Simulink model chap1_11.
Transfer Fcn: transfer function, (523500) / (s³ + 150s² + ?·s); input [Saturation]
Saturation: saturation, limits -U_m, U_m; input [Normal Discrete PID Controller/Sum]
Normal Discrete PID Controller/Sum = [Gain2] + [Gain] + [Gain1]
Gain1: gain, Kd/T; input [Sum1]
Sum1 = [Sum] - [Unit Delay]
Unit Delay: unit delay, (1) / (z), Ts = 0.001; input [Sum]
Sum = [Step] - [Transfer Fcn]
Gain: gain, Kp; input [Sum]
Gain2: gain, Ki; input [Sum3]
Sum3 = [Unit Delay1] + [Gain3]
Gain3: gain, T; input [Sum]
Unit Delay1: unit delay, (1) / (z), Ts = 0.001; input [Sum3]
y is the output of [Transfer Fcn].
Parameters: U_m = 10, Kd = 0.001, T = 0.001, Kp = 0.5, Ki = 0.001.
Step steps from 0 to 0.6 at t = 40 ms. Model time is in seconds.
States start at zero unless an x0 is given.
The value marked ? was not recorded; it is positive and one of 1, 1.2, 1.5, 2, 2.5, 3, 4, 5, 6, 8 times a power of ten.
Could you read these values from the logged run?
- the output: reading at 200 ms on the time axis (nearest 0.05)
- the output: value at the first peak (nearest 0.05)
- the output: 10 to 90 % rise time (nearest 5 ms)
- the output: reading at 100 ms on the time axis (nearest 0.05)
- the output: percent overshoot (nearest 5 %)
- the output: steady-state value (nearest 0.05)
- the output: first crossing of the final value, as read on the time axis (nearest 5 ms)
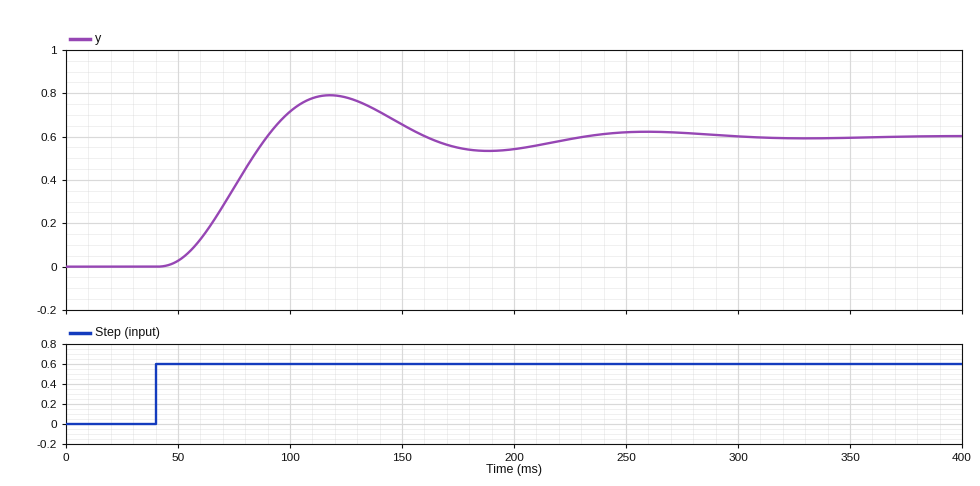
0.55
0.80
30 ms
0.70
30 %
0.60
90 ms
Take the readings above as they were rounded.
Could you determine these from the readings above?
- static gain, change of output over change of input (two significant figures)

1.0
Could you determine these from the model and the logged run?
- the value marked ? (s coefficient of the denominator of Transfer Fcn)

5000
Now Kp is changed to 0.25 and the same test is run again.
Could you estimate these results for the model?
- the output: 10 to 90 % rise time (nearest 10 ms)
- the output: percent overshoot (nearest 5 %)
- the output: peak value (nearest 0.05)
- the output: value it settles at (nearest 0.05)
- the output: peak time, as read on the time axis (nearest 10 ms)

60 ms
10 %
0.65
0.60
160 ms
